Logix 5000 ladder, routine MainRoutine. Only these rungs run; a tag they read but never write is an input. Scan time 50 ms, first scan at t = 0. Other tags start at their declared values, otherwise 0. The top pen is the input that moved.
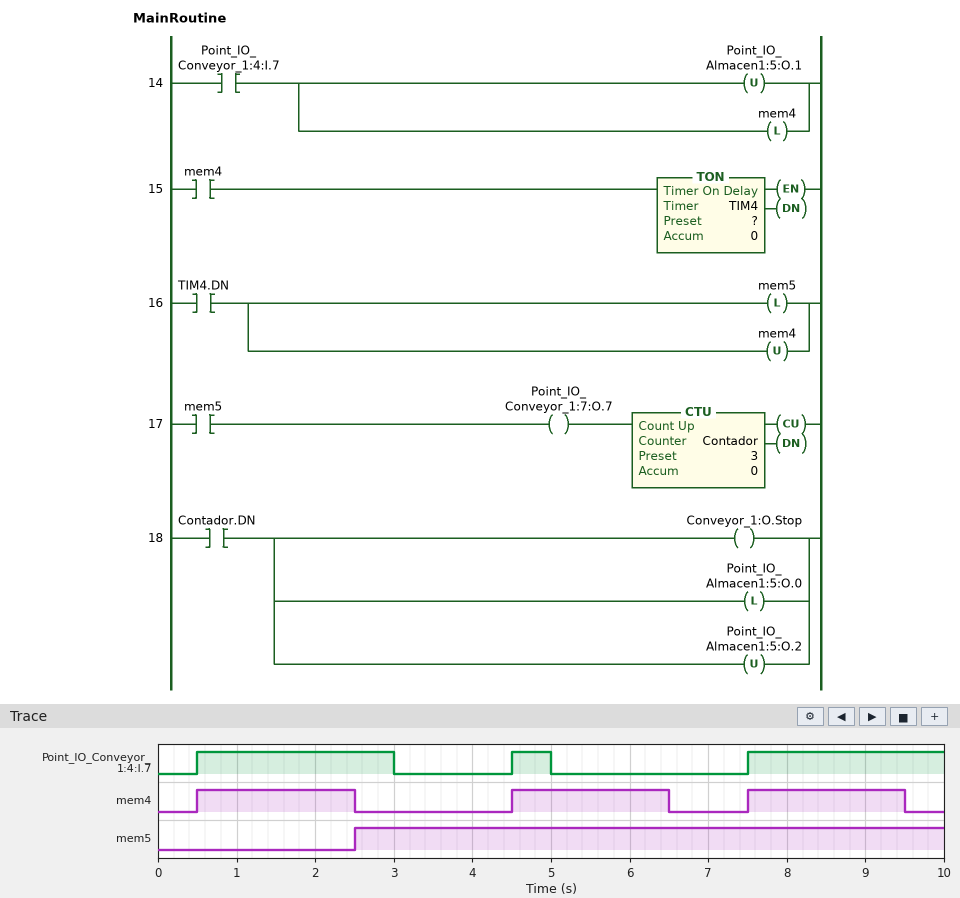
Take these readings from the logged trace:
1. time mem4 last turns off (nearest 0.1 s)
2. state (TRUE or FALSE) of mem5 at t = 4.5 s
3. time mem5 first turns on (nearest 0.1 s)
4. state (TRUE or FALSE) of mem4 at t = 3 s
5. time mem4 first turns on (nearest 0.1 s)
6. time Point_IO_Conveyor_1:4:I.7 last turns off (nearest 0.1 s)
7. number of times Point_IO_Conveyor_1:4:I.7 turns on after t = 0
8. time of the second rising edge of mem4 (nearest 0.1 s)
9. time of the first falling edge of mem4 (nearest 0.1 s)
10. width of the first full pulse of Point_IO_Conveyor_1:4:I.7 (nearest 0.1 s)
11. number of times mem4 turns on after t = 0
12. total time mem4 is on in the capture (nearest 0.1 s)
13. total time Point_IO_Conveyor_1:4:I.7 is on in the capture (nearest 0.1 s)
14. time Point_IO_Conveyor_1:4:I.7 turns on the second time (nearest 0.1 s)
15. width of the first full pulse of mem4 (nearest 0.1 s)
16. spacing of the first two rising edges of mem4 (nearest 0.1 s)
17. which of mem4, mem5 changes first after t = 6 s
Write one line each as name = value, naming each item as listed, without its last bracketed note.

time mem4 last turns off = 9.5 s
state (TRUE or FALSE) of mem5 at t = 4.5 s = TRUE
time mem5 first turns on = 2.5 s
state (TRUE or FALSE) of mem4 at t = 3 s = FALSE
time mem4 first turns on = 0.5 s
time Point_IO_Conveyor_1:4:I.7 last turns off = 5.0 s
number of times Point_IO_Conveyor_1:4:I.7 turns on after t = 0 = 3
time of the second rising edge of mem4 = 4.5 s
time of the first falling edge of mem4 = 2.5 s
width of the first full pulse of Point_IO_Conveyor_1:4:I.7 = 2.5 s
number of times mem4 turns on after t = 0 = 3
total time mem4 is on in the capture = 6.0 s
total time Point_IO_Conveyor_1:4:I.7 is on in the capture = 5.5 s
time Point_IO_Conveyor_1:4:I.7 turns on the second time = 4.5 s
width of the first full pulse of mem4 = 2.0 s
spacing of the first two rising edges of mem4 = 4.0 s
which of mem4, mem5 changes first after t = 6 s = mem4
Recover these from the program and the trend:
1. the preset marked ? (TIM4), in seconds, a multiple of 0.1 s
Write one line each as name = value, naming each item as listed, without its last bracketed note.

the preset marked ? (TIM4), in seconds, a multiple of 0.1 s = 2.0 s
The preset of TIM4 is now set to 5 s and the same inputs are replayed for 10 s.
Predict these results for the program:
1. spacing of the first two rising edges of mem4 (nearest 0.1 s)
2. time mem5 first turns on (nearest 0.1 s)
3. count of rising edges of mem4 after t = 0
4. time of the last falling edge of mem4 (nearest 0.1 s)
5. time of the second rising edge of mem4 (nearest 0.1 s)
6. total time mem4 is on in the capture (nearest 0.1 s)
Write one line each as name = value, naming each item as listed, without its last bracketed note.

spacing of the first two rising edges of mem4 = 7.0 s
time mem5 first turns on = 5.5 s
count of rising edges of mem4 after t = 0 = 2
time of the last falling edge of mem4 = 5.5 s
time of the second rising edge of mem4 = 7.5 s
total time mem4 is on in the capture = 7.5 s
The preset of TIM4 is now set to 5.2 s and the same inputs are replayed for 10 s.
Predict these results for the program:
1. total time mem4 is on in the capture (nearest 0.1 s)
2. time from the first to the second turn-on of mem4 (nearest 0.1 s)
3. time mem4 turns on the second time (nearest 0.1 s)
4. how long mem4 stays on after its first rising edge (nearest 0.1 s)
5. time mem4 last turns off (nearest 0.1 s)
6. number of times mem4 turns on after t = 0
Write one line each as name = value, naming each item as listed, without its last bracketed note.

total time mem4 is on in the capture = 7.7 s
time from the first to the second turn-on of mem4 = 7.0 s
time mem4 turns on the second time = 7.5 s
how long mem4 stays on after its first rising edge = 5.2 s
time mem4 last turns off = 5.7 s
number of times mem4 turns on after t = 0 = 2
